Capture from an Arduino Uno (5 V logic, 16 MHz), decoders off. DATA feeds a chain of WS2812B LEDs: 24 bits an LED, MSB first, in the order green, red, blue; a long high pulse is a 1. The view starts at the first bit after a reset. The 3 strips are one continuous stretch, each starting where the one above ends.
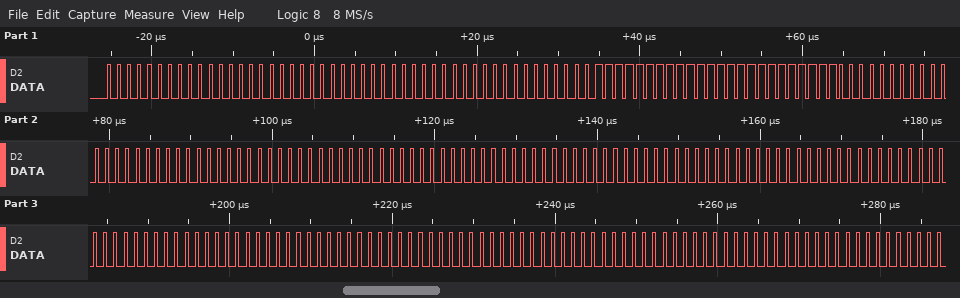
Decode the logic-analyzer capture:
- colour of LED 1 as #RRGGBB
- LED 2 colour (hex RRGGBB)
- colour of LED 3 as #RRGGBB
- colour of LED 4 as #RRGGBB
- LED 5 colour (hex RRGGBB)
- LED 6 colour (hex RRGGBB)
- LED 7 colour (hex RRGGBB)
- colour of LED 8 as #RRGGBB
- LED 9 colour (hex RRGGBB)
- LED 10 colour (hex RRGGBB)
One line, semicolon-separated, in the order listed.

#000000; #000000; #FFFFFF; #000000; #000000; #000000; #000000; #000000; #000000; #000000
